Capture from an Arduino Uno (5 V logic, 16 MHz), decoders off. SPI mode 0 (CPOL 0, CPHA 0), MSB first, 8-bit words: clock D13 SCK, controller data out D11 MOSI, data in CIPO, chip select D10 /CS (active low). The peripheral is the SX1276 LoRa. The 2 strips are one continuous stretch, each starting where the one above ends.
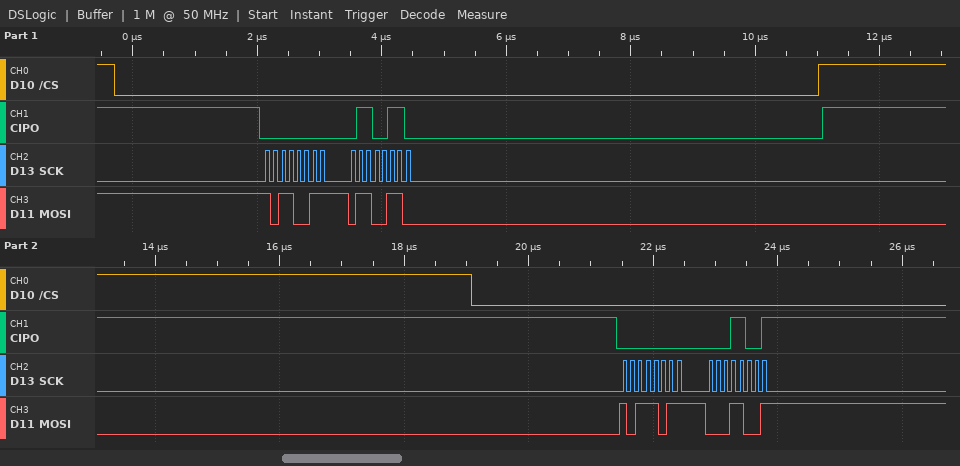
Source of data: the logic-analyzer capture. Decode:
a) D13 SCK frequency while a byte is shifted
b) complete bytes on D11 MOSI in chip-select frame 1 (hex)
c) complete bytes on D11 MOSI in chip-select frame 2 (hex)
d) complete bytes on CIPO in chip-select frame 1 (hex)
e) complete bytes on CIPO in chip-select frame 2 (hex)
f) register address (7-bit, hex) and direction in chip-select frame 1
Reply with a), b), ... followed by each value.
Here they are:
a) 8 MHz
b) 0xB3 0x66
c) 0xBB 0x19
d) 0x00 0x66
e) 0x00 0x19
f) 0x33 write
